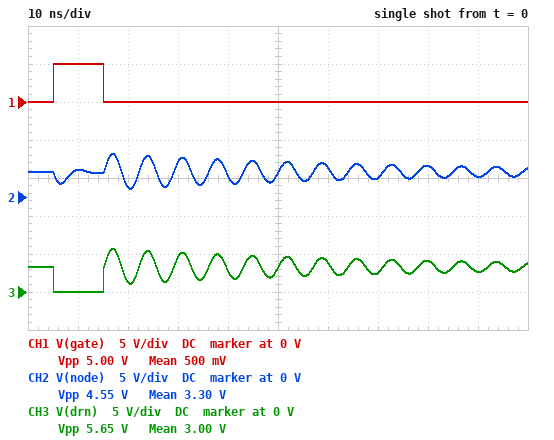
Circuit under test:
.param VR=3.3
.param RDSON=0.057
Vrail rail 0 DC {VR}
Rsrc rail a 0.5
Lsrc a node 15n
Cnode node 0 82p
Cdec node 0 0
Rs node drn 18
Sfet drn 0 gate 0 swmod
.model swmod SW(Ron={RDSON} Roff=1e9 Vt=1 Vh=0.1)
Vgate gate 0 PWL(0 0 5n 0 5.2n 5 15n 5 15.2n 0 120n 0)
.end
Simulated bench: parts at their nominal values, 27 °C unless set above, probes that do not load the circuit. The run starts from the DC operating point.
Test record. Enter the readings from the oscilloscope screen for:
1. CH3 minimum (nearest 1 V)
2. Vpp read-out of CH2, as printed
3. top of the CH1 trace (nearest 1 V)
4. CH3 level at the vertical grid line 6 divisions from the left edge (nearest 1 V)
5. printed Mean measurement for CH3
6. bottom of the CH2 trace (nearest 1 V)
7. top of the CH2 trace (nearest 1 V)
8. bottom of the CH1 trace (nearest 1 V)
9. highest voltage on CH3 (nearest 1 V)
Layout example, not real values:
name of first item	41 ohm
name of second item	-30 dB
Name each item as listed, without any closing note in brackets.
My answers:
CH3 minimum	0 V
Vpp read-out of CH2, as printed	4.55 V
top of the CH1 trace	5 V
CH3 level at the vertical grid line 6 divisions from the left edge	4 V
printed Mean measurement for CH3	3.00 V
bottom of the CH2 trace	1 V
top of the CH2 trace	6 V
bottom of the CH1 trace	0 V
highest voltage on CH3	6 V
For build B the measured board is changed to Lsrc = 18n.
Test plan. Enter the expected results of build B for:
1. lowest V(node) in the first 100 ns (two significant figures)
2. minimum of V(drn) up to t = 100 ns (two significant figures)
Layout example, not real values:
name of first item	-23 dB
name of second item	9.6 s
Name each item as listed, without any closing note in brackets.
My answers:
lowest V(node) in the first 100 ns	910 mV
minimum of V(drn) up to t = 100 ns	5.3 mV
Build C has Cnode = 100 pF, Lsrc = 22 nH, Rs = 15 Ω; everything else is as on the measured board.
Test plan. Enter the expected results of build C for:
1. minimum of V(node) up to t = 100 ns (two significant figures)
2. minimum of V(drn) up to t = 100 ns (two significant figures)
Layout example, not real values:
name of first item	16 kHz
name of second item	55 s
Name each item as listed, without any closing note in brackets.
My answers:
minimum of V(node) up to t = 100 ns	470 mV
minimum of V(drn) up to t = 100 ns	5.7 mV
